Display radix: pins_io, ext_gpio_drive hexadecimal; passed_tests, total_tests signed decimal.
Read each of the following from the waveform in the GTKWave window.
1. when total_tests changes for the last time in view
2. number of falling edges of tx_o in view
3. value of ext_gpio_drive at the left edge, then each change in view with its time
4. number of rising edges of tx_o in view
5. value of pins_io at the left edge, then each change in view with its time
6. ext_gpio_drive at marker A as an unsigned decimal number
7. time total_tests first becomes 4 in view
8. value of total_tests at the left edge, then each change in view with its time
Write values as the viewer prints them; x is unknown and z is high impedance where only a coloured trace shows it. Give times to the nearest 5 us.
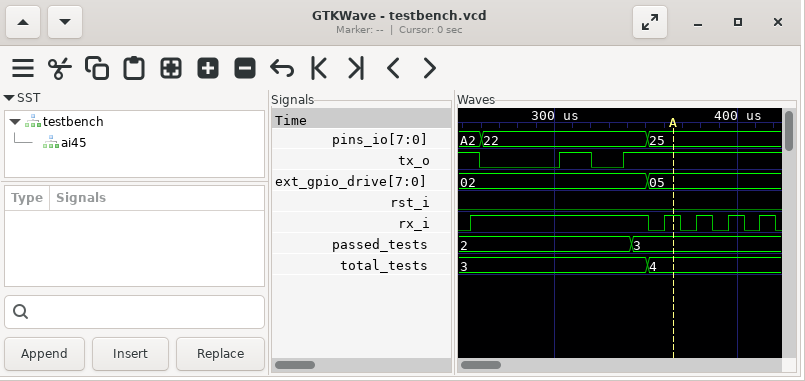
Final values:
350 us
2
02, 05 at 350 us
2
A2, 22 at 260 us, 25 at 350 us
5
350 us
3, 4 at 350 us
